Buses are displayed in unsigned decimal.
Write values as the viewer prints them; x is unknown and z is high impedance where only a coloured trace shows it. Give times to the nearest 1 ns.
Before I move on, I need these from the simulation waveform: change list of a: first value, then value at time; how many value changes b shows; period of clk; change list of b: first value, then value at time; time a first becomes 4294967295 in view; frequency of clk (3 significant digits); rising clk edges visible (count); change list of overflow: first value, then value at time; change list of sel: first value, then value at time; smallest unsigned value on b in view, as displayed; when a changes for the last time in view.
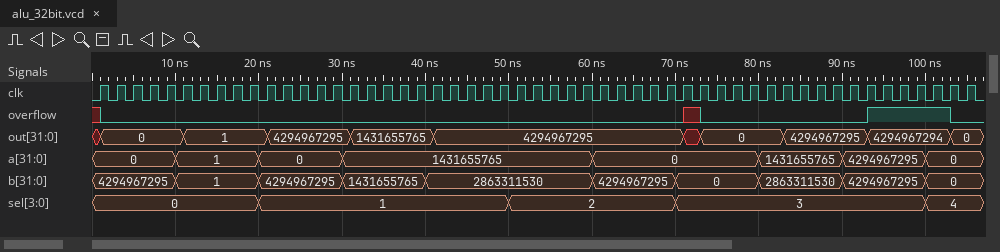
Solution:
0, 1 at 10 ns, 0 at 20 ns, 1431655765 at 30 ns, 0 at 60 ns, 1431655765 at 80 ns, 4294967295 at 90 ns, 0 at 100 ns
9
2 ns
4294967295, 1 at 10 ns, 4294967295 at 20 ns, 1431655765 at 30 ns, 2863311530 at 40 ns, 4294967295 at 60 ns, 0 at 70 ns, 2863311530 at 80 ns, 4294967295 at 90 ns, 0 at 100 ns
90 ns
500 MHz
53
x, 0 at 1 ns, x at 71 ns, 0 at 73 ns, 1 at 93 ns, 0 at 103 ns
0, 1 at 20 ns, 2 at 50 ns, 3 at 70 ns, 4 at 100 ns
0
100 ns
